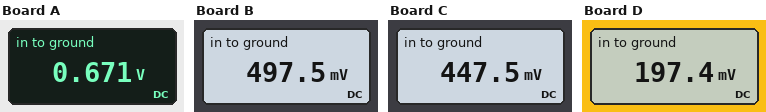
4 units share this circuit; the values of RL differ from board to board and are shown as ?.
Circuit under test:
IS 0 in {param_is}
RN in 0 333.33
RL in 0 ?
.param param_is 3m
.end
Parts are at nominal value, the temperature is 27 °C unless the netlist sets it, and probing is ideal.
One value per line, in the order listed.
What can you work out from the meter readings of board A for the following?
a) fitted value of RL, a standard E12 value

680 Ω
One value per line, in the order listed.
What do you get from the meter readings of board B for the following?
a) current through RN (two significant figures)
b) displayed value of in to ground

1.5 mA
497.5 mV
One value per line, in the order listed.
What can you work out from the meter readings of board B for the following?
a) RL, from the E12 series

330 Ω
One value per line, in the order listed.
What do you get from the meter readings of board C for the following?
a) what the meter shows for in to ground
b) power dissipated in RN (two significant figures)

447.5 mV
600 µW
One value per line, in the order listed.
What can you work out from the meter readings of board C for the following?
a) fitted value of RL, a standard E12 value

270 Ω
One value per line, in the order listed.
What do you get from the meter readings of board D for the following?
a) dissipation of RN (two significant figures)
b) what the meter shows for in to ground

120 µW
197.4 mV
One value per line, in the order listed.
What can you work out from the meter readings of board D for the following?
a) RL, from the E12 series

82 Ω
